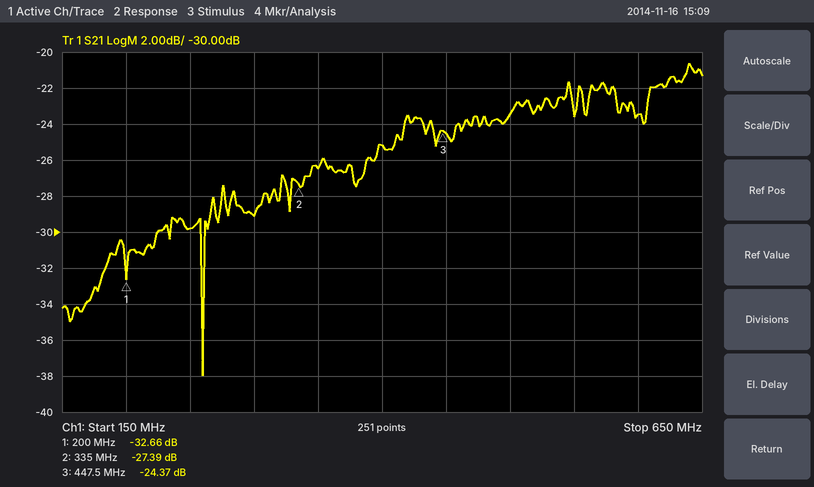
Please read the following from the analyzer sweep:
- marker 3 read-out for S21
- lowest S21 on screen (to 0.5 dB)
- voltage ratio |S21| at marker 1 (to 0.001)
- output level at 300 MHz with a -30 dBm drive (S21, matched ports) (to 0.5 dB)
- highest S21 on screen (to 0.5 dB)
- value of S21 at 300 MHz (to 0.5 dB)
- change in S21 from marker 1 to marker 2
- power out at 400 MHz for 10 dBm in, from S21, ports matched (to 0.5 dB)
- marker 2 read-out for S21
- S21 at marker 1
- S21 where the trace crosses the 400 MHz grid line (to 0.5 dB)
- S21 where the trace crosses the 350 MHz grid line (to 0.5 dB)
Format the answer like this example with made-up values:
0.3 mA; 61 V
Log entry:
-24.37 dB; -38.0 dB; 0.023; -59.0 dBm; -20.5 dB; -29.0 dB; 5.27 dB; -15.0 dBm; -27.39 dB; -32.66 dB; -25.0 dB; -26.5 dB
